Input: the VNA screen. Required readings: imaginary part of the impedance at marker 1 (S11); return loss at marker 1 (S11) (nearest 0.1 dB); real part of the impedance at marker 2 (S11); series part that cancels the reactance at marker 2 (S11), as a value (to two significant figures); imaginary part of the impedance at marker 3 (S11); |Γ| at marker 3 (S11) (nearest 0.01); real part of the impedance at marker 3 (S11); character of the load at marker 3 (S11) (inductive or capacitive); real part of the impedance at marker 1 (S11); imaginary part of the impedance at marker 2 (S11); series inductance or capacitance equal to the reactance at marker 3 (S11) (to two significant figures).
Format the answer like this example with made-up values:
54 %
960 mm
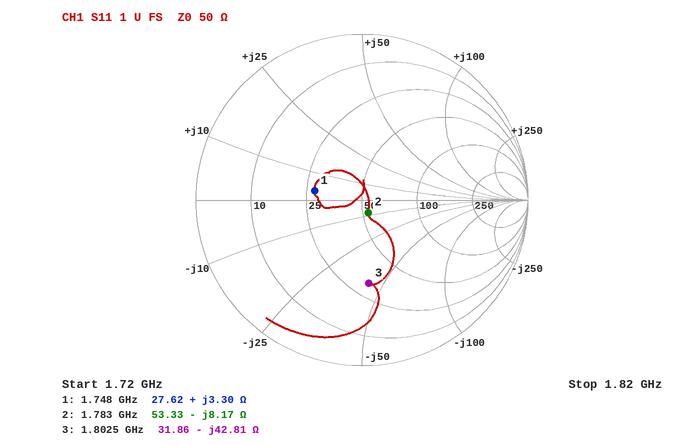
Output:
+3.30 Ω
10.7 dB
53.33 Ω
730 pH
-42.81 Ω
0.50
31.86 Ω
capacitive
27.62 Ω
-8.17 Ω
2.1 pF
